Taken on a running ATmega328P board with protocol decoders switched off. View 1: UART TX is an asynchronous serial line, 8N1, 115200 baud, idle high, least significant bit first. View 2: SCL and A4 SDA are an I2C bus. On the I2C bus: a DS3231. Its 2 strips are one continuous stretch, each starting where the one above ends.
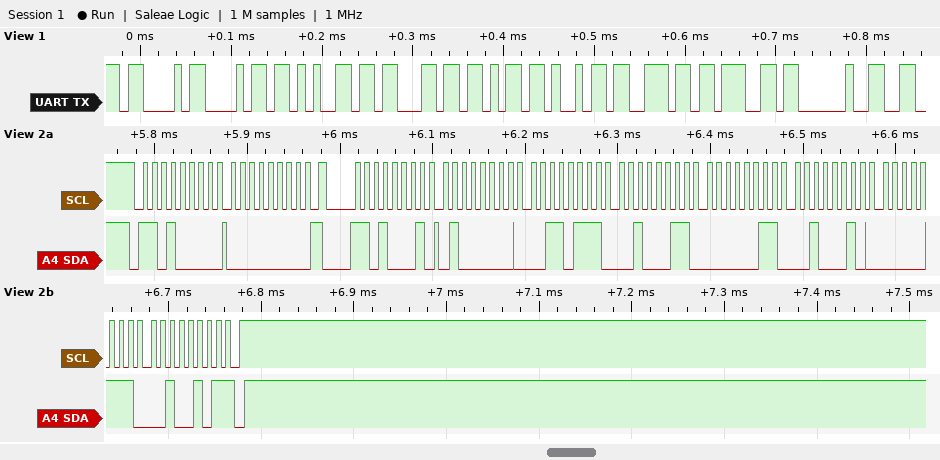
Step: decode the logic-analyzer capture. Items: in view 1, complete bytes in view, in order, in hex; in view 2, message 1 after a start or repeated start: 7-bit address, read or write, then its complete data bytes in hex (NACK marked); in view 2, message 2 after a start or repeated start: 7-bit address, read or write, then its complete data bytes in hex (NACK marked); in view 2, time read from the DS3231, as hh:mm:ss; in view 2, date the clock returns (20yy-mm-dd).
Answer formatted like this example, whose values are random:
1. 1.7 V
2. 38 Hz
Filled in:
1. 43 68 65 63 6B 69 6E 67 20
2. 0x68 write: 00
3. 0x68 read: 40 37 23 03 22 07 25 NACK
4. 23:37:40
5. 2025-07-22
